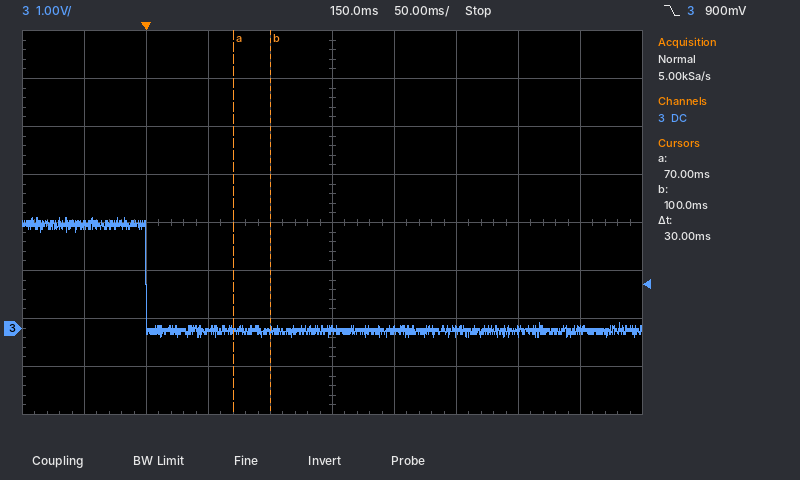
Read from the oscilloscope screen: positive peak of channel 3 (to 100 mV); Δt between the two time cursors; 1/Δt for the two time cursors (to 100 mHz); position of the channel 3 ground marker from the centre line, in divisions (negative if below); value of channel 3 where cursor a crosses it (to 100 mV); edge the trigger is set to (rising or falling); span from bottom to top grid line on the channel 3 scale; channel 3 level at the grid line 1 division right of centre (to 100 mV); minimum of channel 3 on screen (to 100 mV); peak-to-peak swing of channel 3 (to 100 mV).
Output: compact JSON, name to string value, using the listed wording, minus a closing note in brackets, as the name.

{"positive peak of channel 3": "2.3 V", "Δt between the two time cursors": "30 ms", "1/Δt for the two time cursors": "33.3 Hz", "position of the channel 3 ground marker from the centre line, in divisions": "-2.2 div", "value of channel 3 where cursor a crosses it": "0.0 V", "edge the trigger is set to": "falling", "span from bottom to top grid line on the channel 3 scale": "8 V", "channel 3 level at the grid line 1 division right of centre": "0.0 V", "minimum of channel 3 on screen": "-200 mV", "peak-to-peak swing of channel 3": "2.5 V"}
